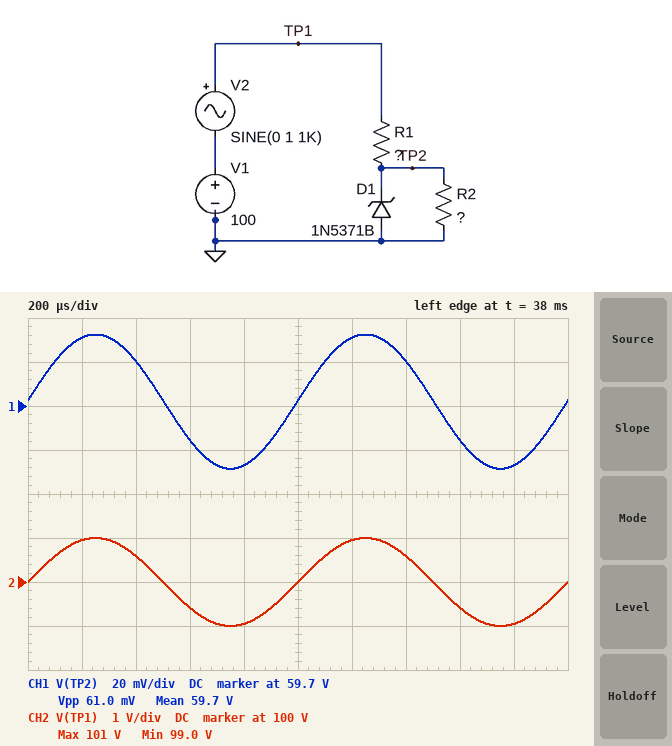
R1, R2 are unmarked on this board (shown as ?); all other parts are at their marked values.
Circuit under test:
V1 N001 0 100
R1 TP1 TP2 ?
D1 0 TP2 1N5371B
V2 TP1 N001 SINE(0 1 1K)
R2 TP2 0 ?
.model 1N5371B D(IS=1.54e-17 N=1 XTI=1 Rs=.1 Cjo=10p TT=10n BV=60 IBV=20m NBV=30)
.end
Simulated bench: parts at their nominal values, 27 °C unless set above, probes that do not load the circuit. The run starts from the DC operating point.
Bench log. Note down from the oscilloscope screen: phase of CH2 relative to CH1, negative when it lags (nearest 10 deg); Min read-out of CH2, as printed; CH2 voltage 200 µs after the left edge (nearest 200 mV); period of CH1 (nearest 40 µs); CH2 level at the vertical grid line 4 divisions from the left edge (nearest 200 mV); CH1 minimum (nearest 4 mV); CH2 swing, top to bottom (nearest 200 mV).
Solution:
0 deg
99.0 V
101.0 V
1.00 ms
99.0 V
59.672 V
2.0 V
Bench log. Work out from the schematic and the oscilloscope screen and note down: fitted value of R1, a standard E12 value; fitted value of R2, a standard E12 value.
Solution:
1.8 kΩ
6.8 kΩ
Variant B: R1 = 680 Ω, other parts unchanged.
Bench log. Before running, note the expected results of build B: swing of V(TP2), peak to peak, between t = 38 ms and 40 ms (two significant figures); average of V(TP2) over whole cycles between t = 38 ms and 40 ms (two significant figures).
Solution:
46 mV
61 V
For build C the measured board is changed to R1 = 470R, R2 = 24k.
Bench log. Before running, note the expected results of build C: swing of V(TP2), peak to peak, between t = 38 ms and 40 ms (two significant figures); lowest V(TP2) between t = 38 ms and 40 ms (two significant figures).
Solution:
41 mV
61 V
